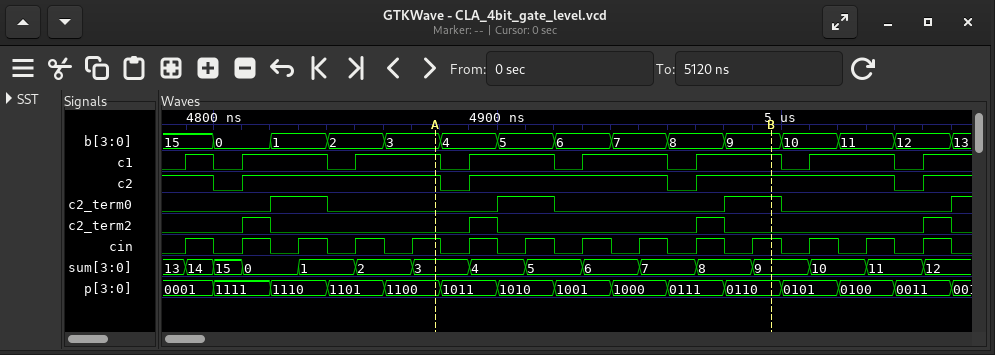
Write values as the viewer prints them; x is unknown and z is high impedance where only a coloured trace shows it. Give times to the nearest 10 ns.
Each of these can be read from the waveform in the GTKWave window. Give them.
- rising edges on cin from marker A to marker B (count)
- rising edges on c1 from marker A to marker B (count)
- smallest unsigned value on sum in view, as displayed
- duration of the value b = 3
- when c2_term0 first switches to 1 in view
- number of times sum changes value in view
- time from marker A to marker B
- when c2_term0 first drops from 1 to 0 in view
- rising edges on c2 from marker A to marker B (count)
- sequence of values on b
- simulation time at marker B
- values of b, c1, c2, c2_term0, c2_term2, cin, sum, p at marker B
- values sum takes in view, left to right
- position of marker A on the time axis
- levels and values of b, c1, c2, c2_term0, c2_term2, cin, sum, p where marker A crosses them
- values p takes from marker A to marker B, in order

6
3
0
20 ns
4820 ns
15
120 ns
4840 ns
2
15, 0, 1, 2, 3, 4, 5, 6, 7, 8, 9, 10, 11, 12, 13
5000 ns
b=9, c1=1, c2=1, c2_term0=1, c2_term2=0, cin=1, sum=9, p=0110
13, 14, 15, 0, 1, 2, 3, 4, 5, 6, 7, 8, 9, 10, 11, 12
4880 ns
b=3, c1=1, c2=1, c2_term0=0, c2_term2=0, cin=1, sum=3, p=1100
1100, 1011, 1010, 1001, 1000, 0111, 0110
